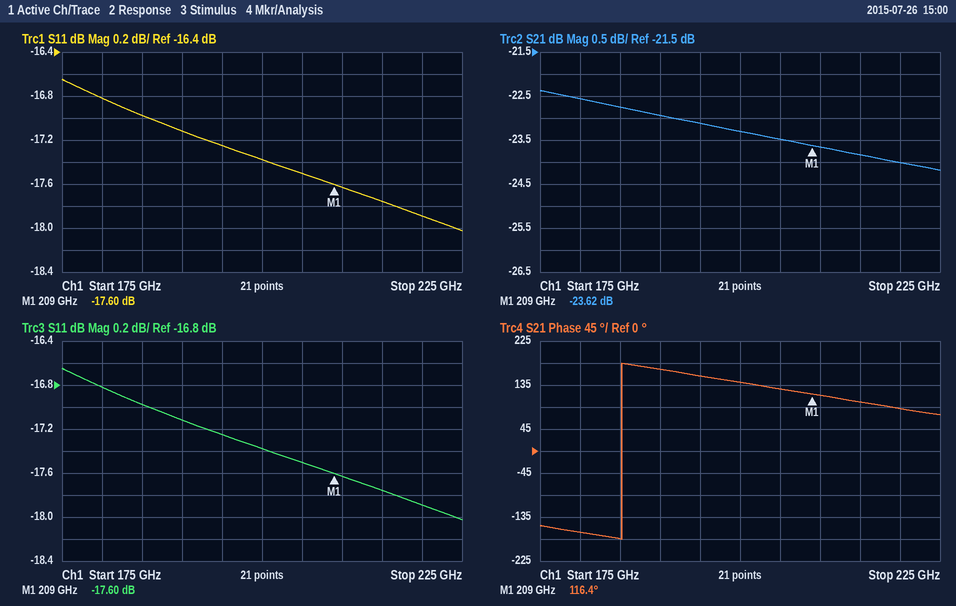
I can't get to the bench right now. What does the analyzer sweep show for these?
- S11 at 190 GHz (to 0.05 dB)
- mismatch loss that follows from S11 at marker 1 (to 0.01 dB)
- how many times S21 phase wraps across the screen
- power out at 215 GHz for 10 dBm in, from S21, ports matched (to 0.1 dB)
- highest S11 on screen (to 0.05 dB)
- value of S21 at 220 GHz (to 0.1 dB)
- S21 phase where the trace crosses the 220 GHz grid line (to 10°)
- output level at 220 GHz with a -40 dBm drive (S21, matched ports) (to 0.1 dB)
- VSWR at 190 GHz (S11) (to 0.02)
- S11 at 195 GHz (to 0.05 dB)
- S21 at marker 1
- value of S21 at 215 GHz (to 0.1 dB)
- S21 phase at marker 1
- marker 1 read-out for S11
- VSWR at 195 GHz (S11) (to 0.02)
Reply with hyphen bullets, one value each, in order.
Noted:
- -17.10 dB
- 0.08 dB
- 1
- -13.8 dBm
- -16.65 dB
- -24.0 dB
- 90°
- -64.0 dBm
- 1.32
- -17.25 dB
- -23.62 dB
- -23.8 dB
- 116.4°
- -17.60 dB
- 1.32
